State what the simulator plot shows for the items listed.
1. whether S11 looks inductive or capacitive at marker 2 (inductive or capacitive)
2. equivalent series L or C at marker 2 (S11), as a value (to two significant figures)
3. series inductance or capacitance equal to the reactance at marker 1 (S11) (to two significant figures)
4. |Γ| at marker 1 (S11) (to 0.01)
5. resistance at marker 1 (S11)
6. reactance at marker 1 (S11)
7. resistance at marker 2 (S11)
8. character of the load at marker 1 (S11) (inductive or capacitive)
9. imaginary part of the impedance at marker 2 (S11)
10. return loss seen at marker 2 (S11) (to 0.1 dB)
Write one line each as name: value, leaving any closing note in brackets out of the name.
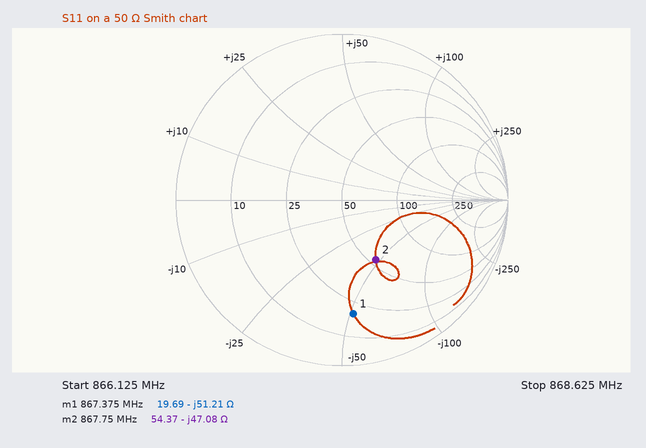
whether S11 looks inductive or capacitive at marker 2: capacitive
equivalent series L or C at marker 2 (S11), as a value: 3.9 pF
series inductance or capacitance equal to the reactance at marker 1 (S11): 3.6 pF
|Γ| at marker 1 (S11): 0.69
resistance at marker 1: 19.69 Ω
reactance at marker 1: -51.21 Ω
resistance at marker 2: 54.37 Ω
character of the load at marker 1 (S11): capacitive
imaginary part of the impedance at marker 2: -47.08 Ω
return loss seen at marker 2 (S11): 7.7 dB
